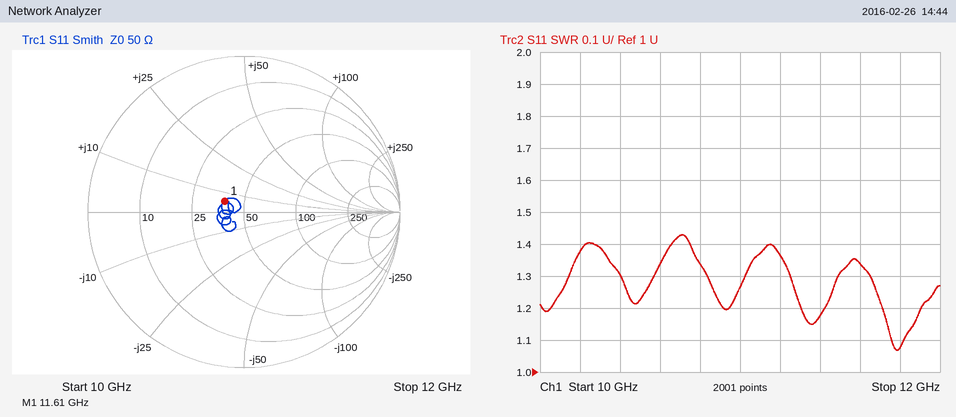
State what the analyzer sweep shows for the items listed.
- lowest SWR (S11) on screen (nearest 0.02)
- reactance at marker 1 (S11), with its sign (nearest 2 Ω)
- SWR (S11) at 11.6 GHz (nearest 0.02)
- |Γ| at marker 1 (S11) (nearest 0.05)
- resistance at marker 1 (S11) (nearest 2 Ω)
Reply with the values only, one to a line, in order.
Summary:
1.06
+6 Ω
1.34
0.15
38 Ω
